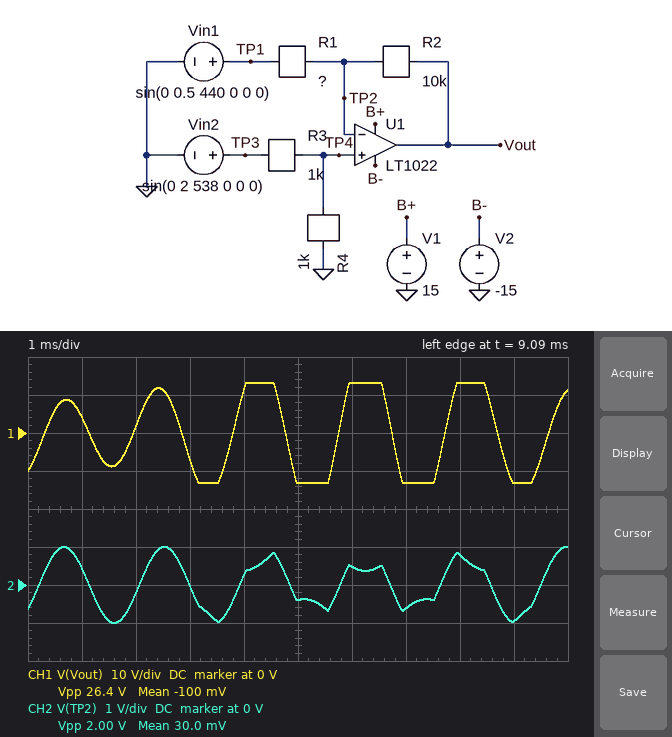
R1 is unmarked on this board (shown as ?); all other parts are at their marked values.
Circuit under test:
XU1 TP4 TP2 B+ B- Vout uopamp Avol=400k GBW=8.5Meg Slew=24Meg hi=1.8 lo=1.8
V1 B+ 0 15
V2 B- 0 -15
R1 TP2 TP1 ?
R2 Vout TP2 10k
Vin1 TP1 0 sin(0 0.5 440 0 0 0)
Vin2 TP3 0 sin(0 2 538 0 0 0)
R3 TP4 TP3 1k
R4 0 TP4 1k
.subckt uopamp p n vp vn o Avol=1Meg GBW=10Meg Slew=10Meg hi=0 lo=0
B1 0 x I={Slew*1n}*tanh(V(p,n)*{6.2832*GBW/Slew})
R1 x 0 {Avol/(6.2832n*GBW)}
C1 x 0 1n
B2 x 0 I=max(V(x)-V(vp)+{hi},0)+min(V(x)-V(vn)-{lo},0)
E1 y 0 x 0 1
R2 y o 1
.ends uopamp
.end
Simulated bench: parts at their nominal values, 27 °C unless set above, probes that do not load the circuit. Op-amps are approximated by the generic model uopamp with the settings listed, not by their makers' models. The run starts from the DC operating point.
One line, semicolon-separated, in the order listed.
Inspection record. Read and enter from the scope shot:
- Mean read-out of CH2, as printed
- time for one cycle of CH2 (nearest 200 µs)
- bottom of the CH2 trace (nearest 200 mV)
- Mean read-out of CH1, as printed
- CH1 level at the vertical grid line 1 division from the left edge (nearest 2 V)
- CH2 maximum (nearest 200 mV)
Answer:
30.0 mV; 1.8 ms; -1.0 V; -100 mV; 4 V; 1.0 V
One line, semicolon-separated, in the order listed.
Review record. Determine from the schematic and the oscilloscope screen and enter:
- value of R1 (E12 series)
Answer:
680 Ω
